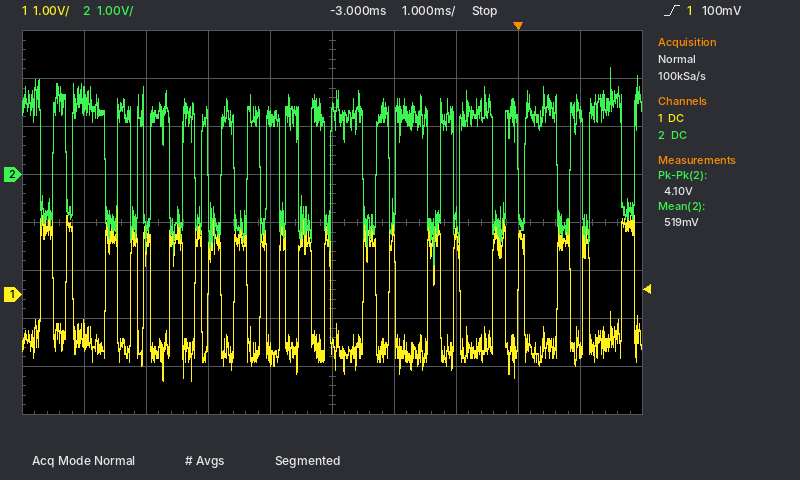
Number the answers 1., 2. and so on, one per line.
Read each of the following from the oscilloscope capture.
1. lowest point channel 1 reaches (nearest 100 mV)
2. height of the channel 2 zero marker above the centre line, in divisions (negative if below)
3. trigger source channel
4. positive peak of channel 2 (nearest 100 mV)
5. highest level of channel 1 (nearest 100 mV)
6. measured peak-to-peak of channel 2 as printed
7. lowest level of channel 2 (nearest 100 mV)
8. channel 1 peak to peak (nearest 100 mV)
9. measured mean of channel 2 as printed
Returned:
1. -1.8 V
2. +1.0 div
3. channel 1
4. 2.2 V
5. 1.8 V
6. 4.10 V
7. -1.9 V
8. 3.6 V
9. 519 mV
